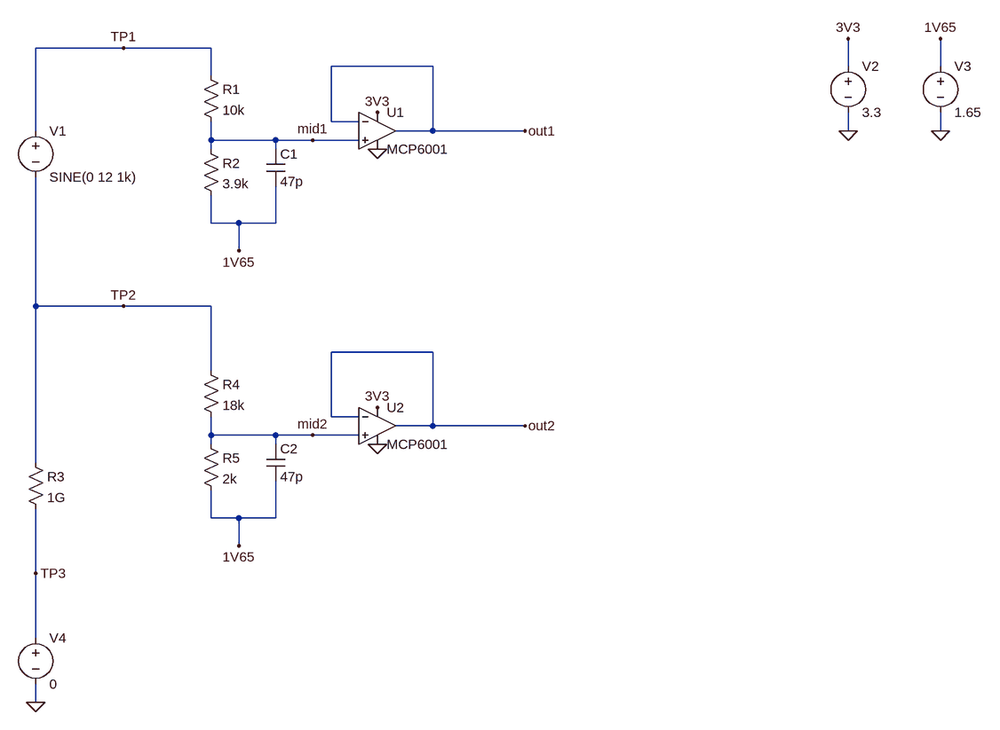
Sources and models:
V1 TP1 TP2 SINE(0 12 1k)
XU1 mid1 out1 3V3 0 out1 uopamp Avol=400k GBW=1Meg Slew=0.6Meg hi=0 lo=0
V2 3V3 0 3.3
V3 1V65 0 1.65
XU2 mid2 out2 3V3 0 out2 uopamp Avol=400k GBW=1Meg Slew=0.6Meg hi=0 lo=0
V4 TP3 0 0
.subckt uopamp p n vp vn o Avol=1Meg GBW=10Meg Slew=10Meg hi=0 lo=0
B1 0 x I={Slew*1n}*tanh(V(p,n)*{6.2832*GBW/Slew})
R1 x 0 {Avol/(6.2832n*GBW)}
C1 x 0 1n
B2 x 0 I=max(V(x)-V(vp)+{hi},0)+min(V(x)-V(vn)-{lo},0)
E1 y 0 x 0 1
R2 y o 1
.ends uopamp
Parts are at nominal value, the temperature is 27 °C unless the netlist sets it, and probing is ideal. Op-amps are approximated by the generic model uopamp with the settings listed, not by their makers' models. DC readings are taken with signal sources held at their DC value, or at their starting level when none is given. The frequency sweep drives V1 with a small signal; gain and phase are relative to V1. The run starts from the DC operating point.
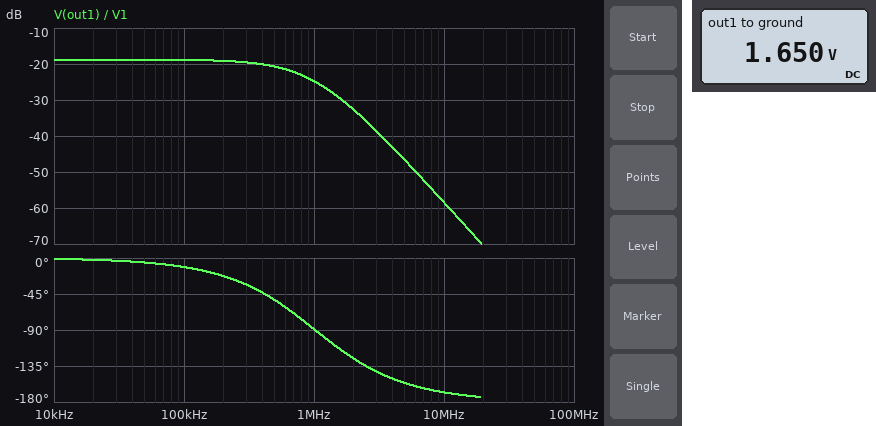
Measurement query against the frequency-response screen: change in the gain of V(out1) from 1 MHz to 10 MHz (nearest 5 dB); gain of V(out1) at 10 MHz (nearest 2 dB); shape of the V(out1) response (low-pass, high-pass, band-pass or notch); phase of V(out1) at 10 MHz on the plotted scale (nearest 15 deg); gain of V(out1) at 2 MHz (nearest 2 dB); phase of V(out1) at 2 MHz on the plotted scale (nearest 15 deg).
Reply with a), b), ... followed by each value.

a) -35 dB
b) -58 dB
c) low-pass
d) -165 deg
e) -32 dB
f) -120 deg
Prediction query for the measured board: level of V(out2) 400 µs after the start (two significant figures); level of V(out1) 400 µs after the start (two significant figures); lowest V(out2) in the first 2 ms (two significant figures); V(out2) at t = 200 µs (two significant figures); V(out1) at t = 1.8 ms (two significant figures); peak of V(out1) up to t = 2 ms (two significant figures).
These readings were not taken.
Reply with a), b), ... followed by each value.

a) 1.2 V
b) 2.5 V
c) 940 mV
d) 980 mV
e) 340 mV
f) 3.0 V
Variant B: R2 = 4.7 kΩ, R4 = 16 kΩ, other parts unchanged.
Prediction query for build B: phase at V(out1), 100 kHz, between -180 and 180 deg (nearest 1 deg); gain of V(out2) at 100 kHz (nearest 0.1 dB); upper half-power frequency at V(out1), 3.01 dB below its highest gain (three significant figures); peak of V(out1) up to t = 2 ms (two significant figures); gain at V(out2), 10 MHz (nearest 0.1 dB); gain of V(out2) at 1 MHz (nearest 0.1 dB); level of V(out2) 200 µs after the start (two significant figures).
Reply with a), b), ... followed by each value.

a) -12 deg
b) -24.3 dB
c) 593 kHz
d) 3.3 V
e) -57.9 dB
f) -27.6 dB
g) 950 mV
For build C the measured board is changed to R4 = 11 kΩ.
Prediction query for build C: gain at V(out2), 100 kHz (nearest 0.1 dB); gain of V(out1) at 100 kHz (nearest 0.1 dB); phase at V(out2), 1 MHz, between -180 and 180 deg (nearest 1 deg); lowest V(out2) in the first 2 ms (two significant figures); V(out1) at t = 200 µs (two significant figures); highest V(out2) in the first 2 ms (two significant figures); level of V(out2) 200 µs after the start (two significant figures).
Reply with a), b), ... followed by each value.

a) -22.6 dB
b) -16.9 dB
c) 111 deg
d) 760 mV
e) 3.3 V
f) 2.5 V
g) 800 mV
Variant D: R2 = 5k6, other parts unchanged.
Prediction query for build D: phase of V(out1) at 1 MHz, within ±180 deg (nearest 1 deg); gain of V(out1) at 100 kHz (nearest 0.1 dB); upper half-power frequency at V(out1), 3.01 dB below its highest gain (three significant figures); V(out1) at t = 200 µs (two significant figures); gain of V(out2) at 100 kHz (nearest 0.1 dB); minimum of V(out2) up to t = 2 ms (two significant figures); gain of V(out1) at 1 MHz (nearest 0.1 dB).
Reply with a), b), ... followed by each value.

a) -98 deg
b) -16.2 dB
c) 538 kHz
d) 3.3 V
e) -25.0 dB
f) 980 mV
g) -23.6 dB
